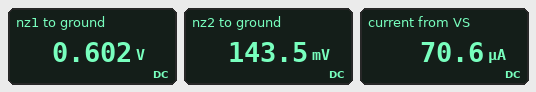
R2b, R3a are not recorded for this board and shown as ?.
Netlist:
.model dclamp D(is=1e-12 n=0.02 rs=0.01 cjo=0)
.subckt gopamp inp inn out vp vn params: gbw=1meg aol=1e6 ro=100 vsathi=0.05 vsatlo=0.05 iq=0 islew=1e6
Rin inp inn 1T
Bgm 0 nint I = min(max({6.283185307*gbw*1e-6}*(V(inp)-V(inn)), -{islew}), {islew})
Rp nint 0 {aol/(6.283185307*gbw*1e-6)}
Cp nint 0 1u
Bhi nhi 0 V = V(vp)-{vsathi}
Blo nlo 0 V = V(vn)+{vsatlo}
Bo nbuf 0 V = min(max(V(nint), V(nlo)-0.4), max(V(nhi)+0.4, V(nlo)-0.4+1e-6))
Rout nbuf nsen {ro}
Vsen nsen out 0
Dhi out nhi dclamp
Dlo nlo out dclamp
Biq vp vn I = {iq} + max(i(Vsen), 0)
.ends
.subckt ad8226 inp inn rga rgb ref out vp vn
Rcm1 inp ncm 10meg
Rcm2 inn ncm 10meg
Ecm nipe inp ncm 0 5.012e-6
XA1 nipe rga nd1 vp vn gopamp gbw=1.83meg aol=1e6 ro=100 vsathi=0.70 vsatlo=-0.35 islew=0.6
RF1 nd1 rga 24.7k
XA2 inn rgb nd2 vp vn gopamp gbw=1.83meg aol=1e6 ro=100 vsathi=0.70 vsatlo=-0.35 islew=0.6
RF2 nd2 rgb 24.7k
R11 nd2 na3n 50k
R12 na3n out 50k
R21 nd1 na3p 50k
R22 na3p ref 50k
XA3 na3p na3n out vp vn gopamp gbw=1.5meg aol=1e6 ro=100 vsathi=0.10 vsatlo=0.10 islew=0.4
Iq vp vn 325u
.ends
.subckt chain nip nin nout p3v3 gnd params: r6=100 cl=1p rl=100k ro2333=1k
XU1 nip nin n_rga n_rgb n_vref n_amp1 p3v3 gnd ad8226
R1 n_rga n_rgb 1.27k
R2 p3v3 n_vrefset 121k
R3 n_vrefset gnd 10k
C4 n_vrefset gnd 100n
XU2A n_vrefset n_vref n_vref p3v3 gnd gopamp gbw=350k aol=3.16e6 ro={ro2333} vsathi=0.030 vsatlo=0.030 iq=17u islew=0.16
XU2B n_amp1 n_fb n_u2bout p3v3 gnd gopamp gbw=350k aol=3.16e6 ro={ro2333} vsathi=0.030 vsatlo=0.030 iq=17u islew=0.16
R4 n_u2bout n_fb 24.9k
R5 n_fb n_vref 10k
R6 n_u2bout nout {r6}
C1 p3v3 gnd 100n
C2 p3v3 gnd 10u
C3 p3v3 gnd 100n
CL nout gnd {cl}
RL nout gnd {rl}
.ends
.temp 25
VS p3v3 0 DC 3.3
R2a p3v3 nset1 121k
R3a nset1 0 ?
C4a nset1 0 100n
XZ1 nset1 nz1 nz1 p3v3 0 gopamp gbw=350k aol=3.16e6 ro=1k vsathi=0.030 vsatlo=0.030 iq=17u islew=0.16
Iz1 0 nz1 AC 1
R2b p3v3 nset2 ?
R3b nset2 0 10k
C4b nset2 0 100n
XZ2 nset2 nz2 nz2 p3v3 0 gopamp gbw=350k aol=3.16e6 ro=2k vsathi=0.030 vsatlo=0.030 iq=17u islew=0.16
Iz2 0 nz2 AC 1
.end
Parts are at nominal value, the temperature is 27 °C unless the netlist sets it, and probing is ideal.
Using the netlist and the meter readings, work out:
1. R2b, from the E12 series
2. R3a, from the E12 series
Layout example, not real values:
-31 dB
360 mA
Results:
220 kΩ
27 kΩ
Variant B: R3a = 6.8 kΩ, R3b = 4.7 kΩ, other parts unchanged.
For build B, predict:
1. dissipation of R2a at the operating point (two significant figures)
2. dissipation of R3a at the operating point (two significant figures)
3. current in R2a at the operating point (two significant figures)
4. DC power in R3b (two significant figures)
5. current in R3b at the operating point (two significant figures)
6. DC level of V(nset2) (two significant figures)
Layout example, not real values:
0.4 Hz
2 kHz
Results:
81 µW
4.5 µW
26 µA
1.0 µW
15 µA
69 mV
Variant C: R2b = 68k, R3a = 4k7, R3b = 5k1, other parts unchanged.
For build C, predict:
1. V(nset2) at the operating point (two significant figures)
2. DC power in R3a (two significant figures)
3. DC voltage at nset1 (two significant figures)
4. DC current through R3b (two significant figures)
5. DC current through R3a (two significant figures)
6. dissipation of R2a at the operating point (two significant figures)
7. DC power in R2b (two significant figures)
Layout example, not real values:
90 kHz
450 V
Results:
230 mV
3.2 µW
120 mV
45 µA
26 µA
83 µW
140 µW
